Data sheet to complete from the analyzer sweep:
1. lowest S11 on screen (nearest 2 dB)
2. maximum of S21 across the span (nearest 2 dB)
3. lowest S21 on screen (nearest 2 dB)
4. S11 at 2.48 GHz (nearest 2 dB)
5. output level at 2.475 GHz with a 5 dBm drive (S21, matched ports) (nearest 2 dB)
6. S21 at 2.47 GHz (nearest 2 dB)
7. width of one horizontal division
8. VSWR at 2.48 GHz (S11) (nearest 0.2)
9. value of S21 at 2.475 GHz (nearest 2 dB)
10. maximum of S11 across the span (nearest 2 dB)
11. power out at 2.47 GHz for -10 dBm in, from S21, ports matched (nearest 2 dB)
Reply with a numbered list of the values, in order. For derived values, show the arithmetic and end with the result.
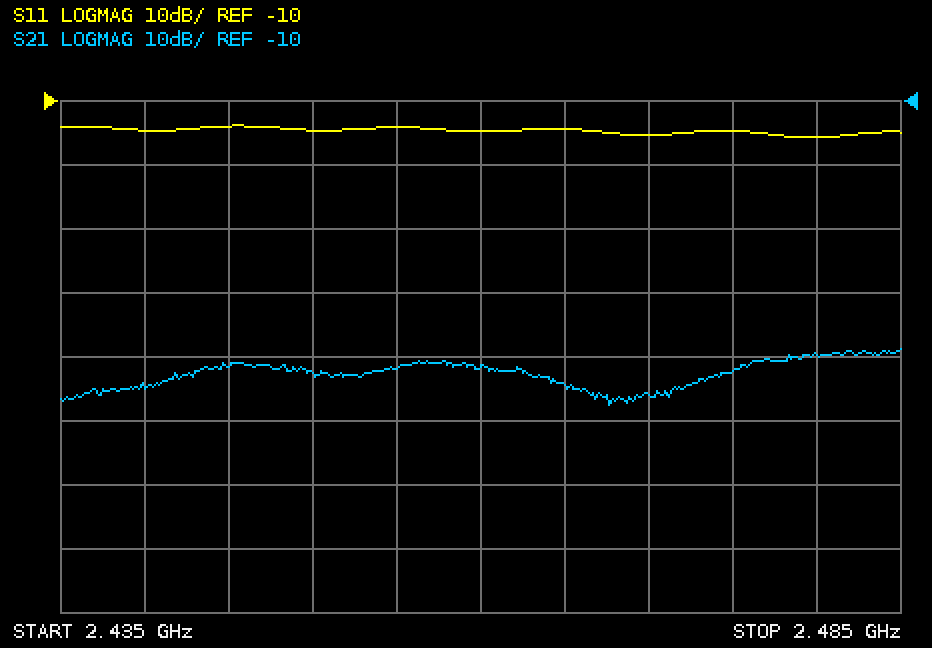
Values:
1. -16 dB
2. -48 dB
3. -58 dB
4. -16 dB
5. 5 dBm + (-52 dB) = -48 dBm
6. -56 dB
7. 5 MHz
8. |Γ| = 10^(-16/20) = 0.1585; VSWR = (1 + 0.1585)/(1 − 0.1585) ≈ 1.4
9. -52 dB
10. -14 dB
11. -10 dBm + (-56 dB) = -66 dBm
